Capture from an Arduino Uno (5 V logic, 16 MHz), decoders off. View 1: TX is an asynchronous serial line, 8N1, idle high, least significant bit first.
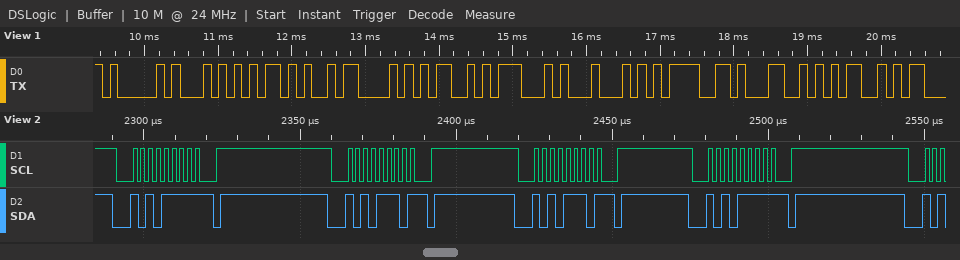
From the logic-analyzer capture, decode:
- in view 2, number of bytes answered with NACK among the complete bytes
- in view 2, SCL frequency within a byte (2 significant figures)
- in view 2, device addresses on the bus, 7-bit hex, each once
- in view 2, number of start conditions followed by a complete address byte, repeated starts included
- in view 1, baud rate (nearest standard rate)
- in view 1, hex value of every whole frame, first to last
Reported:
4
400 kHz
0x57
4
9600 baud
0x41 0x54 0x2B 0x43 0x4D 0x47 0x44 0x3D 0x31 0x35
